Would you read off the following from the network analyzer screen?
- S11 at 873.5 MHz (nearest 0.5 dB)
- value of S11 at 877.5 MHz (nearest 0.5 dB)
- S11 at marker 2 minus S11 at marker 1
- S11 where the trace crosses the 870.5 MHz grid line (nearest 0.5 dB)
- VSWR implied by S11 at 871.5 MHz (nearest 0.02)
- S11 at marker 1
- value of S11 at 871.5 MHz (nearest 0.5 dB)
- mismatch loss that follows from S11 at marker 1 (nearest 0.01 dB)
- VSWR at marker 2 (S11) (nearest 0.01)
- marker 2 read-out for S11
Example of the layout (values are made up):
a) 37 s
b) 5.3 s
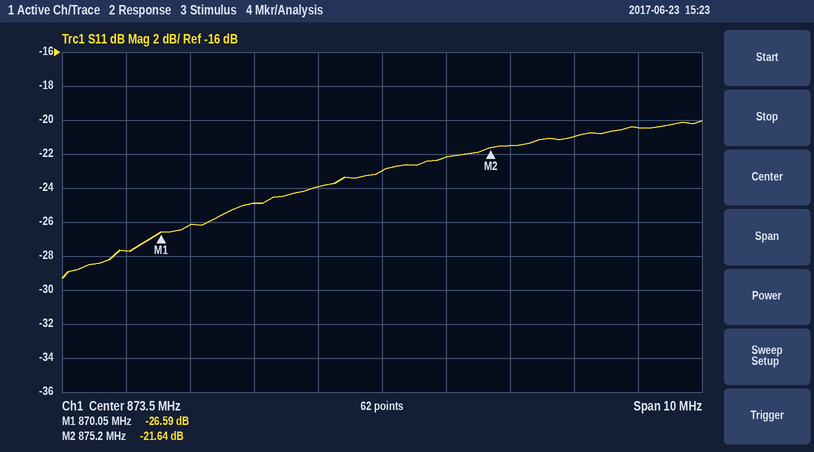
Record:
a) -23.0 dB
b) -20.5 dB
c) 4.95 dB
d) -26.0 dB
e) 1.12
f) -26.59 dB
g) -25.0 dB
h) 0.01 dB
i) 1.18
j) -21.64 dB
